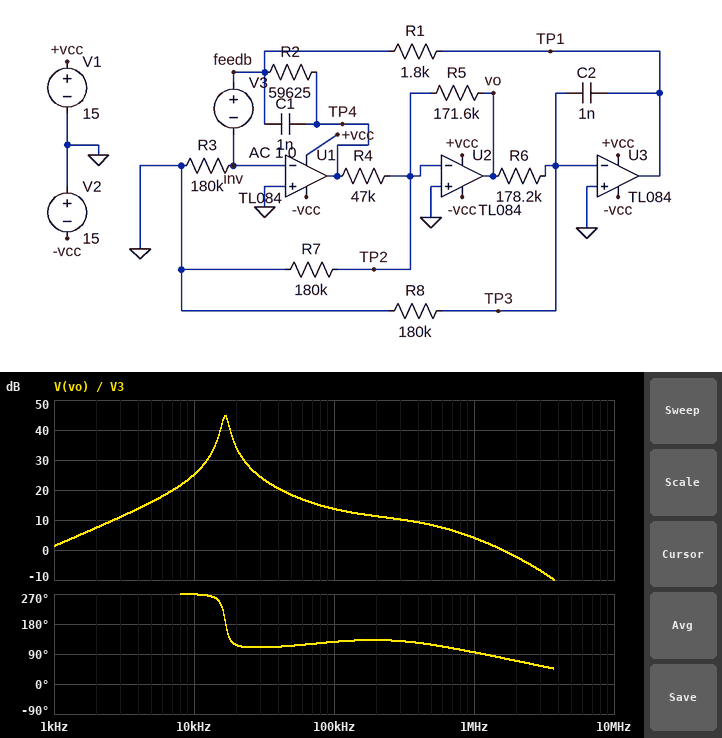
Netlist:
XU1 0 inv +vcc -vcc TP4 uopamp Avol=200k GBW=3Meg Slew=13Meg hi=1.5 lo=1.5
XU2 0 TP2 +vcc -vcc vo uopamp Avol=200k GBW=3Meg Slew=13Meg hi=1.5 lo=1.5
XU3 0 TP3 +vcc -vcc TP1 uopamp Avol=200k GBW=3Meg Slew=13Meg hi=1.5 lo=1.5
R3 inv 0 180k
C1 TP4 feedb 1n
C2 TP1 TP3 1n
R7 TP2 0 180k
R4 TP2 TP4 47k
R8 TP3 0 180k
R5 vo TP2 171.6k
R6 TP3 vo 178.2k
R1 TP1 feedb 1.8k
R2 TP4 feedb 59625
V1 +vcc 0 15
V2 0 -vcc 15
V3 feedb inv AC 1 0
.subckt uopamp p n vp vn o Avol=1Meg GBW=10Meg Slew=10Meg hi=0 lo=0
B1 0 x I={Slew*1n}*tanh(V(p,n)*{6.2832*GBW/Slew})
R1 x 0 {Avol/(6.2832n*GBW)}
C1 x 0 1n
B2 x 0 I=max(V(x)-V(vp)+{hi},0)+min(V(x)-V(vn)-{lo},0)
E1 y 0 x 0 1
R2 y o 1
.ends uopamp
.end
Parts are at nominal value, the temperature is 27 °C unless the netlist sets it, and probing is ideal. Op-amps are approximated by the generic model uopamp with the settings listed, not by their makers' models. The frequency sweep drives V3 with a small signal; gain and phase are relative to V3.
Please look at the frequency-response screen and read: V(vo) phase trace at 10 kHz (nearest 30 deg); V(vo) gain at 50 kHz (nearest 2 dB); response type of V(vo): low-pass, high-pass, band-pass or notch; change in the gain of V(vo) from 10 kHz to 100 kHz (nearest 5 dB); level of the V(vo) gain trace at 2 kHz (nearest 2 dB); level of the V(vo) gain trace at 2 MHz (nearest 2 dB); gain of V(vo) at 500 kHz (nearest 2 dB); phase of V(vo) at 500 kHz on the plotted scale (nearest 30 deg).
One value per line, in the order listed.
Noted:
270 deg
18 dB
band-pass
-10 dB
8 dB
-2 dB
8 dB
120 deg
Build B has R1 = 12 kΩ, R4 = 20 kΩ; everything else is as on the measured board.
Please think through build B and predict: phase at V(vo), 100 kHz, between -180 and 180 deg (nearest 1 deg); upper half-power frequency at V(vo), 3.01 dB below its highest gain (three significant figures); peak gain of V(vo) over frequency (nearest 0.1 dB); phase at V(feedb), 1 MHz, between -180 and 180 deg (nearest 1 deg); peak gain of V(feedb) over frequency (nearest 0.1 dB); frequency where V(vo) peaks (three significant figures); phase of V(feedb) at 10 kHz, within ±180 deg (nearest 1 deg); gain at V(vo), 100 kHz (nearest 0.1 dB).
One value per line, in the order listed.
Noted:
151 deg
11.3 kHz
37.1 dB
-18 deg
0.2 dB
10.1 kHz
-1 deg
18.3 dB
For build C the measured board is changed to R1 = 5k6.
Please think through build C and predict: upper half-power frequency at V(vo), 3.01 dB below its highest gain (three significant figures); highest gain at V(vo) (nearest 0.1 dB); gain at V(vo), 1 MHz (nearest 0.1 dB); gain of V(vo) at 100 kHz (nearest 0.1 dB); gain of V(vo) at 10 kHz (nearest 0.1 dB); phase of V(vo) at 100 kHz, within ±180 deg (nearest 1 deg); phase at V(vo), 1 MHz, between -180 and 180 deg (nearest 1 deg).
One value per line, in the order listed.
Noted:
10.9 kHz
33.8 dB
4.2 dB
11.5 dB
33.3 dB
152 deg
98 deg
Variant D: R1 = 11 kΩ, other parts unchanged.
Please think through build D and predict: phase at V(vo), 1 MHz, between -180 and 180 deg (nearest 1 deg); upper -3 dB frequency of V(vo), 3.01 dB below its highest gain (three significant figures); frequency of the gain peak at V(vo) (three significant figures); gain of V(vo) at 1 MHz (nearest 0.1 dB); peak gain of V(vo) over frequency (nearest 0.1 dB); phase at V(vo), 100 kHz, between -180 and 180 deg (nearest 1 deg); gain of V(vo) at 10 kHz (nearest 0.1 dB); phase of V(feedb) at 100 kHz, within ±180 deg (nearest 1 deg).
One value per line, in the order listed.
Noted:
99 deg
8.33 kHz
6.88 kHz
4.2 dB
28.4 dB
159 deg
21.8 dB
-2 deg
